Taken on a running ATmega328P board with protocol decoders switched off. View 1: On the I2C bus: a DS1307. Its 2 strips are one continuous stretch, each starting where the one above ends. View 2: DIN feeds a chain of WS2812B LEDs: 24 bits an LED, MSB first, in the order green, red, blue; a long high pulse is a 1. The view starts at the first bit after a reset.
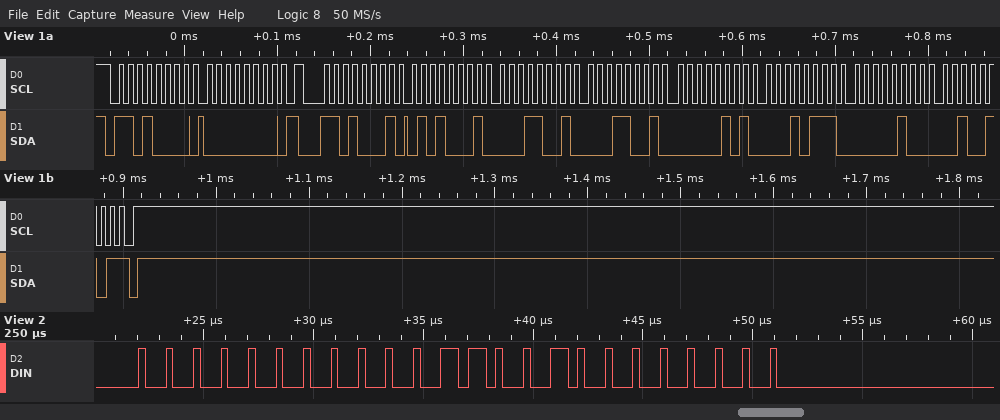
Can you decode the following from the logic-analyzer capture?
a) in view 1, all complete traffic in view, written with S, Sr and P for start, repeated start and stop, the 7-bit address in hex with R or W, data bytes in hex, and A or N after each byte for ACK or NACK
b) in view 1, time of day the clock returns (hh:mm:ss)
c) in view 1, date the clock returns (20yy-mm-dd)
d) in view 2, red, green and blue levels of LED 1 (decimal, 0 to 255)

S 68W A 00 A Sr 68R A 51 A 19 A 19 A 05 A 17 A 04 A 25 N P
19:19:51
2025-04-17
25, 0, 0
